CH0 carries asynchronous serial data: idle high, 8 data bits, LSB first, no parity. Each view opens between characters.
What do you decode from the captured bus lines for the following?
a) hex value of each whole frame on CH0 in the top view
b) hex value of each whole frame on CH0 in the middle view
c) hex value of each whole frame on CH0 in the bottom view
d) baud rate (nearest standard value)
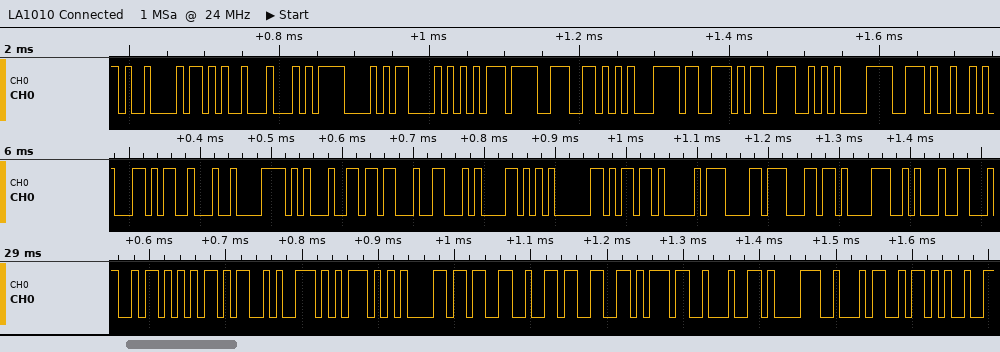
09, 2B, 44, 0F, 0D, D5, CF, 56, BC, AE, 4E, E1, 2E
AC, 22, 78, 91, 1B, 46, 58, 81, 6D, D0, D8, 6C, 38, 91
5A, AD, CA, 75, 85, 9B, B2, 66, 37, 64, 38, 34, 2B
115200 baud
